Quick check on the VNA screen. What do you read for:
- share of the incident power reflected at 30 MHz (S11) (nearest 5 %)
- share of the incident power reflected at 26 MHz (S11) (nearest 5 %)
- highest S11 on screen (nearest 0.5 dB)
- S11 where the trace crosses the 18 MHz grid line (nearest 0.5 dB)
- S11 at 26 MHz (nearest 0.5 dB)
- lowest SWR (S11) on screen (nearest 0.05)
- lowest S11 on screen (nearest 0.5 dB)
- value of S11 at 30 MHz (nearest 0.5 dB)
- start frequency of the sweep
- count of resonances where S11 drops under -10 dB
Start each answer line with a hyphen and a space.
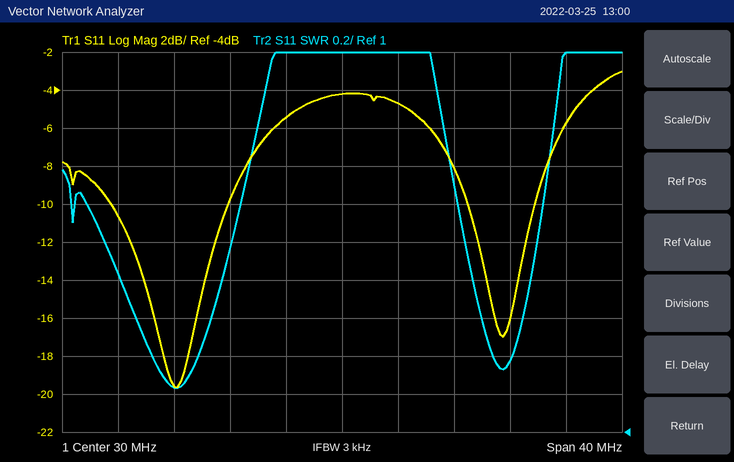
- 40 %
- 30 %
- -3.0 dB
- -19.5 dB
- -5.5 dB
- 1.25
- -19.5 dB
- -4.0 dB
- 10 MHz
- 2
